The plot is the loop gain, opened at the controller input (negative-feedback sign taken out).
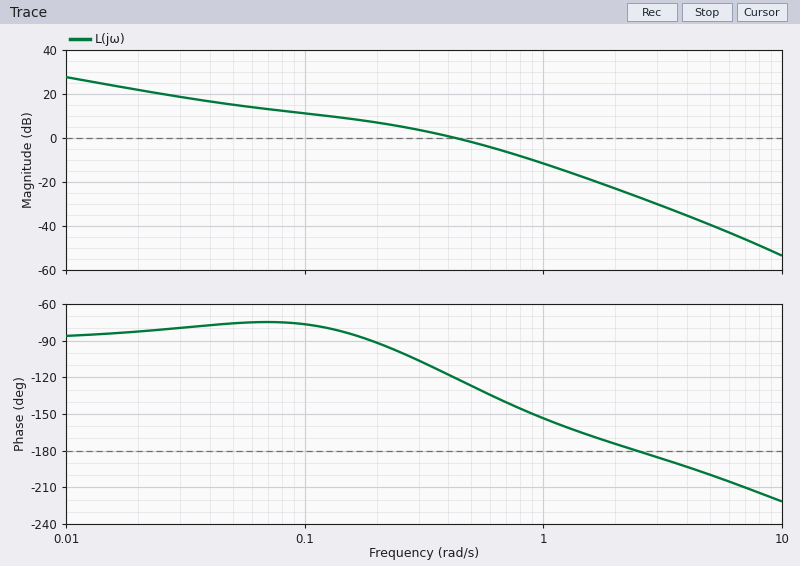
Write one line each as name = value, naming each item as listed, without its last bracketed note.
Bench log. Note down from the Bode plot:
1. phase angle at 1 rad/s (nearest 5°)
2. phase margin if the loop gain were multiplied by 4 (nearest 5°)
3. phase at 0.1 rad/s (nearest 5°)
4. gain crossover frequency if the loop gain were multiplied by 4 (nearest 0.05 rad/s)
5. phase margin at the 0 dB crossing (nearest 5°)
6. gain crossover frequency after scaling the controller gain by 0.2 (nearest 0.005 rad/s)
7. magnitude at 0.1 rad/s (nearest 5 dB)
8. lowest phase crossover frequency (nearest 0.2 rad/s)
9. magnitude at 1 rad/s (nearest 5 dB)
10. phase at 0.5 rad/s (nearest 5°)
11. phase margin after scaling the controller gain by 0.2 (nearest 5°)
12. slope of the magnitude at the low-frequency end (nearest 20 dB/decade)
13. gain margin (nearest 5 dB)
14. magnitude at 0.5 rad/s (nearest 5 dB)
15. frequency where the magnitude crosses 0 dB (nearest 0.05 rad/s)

phase angle at 1 rad/s = -155°
phase margin if the loop gain were multiplied by 4 = 25°
phase at 0.1 rad/s = -75°
gain crossover frequency if the loop gain were multiplied by 4 = 1.05 rad/s
phase margin at the 0 dB crossing = 60°
gain crossover frequency after scaling the controller gain by 0.2 = 0.060 rad/s
magnitude at 0.1 rad/s = 10 dB
lowest phase crossover frequency = 2.4 rad/s
magnitude at 1 rad/s = -10 dB
phase at 0.5 rad/s = -125°
phase margin after scaling the controller gain by 0.2 = 105°
slope of the magnitude at the low-frequency end = -20 dB/decade
gain margin = 25 dB
magnitude at 0.5 rad/s = 0 dB
frequency where the magnitude crosses 0 dB = 0.45 rad/s
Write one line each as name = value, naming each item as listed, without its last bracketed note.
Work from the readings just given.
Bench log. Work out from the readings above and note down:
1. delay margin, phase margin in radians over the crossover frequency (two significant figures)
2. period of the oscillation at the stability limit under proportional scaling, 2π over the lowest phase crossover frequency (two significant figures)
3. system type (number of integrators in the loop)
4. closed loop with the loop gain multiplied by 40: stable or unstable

delay margin, phase margin in radians over the crossover frequency = 2.3 s
period of the oscillation at the stability limit under proportional scaling, 2π over the lowest phase crossover frequency = 2.6 s
system type = 1
closed loop with the loop gain multiplied by 40: stable or unstable = unstable
